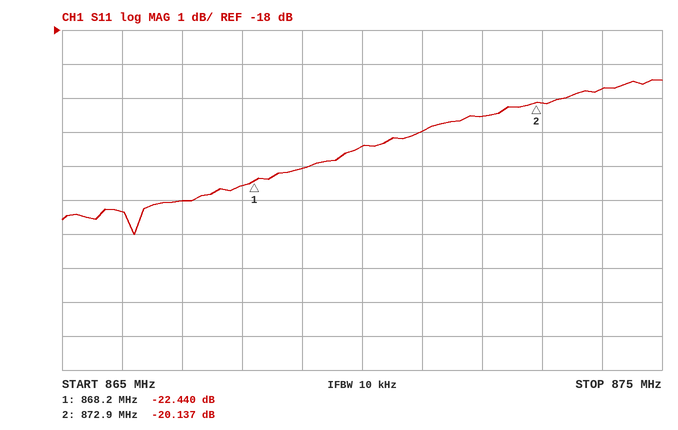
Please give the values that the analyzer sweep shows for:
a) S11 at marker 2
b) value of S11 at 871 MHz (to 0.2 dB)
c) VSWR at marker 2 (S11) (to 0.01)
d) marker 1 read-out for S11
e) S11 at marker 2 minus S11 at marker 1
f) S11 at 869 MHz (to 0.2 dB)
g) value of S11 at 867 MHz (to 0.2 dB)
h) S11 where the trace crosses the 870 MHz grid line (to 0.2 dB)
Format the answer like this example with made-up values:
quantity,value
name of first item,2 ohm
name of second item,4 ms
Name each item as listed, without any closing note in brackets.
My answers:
quantity,value
S11 at marker 2,-20.137 dB
value of S11 at 871 MHz,-21.0 dB
VSWR at marker 2 (S11),1.22
marker 1 read-out for S11,-22.440 dB
S11 at marker 2 minus S11 at marker 1,2.303 dB
S11 at 869 MHz,-22.0 dB
value of S11 at 867 MHz,-23.0 dB
S11 where the trace crosses the 870 MHz grid line,-21.4 dB
